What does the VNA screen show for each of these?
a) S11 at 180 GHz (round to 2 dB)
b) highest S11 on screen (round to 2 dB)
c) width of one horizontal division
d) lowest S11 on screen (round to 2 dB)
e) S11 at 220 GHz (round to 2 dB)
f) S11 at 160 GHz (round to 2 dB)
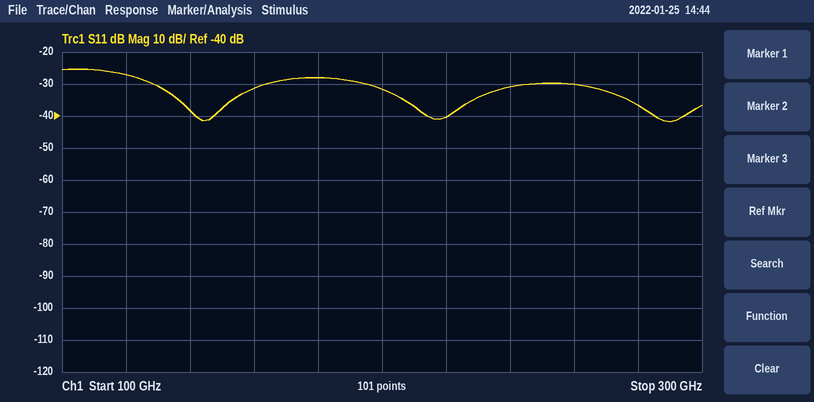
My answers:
-28 dB
-26 dB
20 GHz
-42 dB
-40 dB
-32 dB
